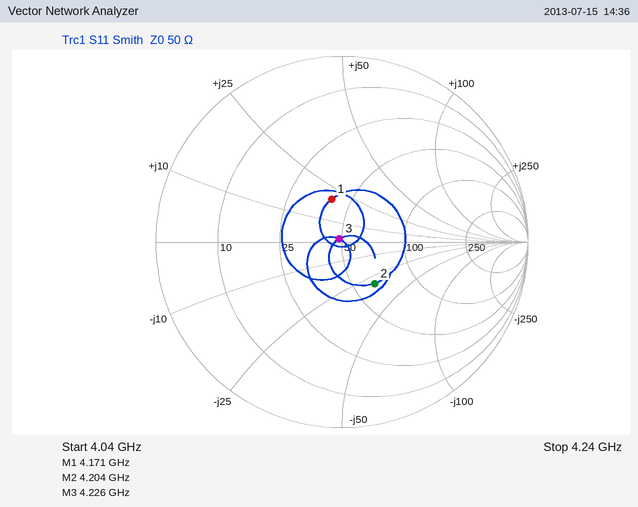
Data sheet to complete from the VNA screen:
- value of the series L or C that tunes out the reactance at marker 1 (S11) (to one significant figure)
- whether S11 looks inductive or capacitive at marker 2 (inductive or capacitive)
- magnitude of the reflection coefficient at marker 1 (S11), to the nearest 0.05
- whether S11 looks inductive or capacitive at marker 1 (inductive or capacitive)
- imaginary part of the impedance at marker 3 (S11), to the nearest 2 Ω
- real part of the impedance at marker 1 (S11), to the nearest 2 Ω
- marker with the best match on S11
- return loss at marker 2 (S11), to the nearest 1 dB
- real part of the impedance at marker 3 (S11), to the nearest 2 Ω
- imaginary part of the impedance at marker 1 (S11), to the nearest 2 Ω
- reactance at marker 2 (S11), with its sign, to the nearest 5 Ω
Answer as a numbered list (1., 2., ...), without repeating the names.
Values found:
1. 2 pF
2. capacitive
3. 0.25
4. inductive
5. +2 Ω
6. 40 Ω
7. marker 3
8. 11 dB
9. 48 Ω
10. +20 Ω
11. -30 Ω
